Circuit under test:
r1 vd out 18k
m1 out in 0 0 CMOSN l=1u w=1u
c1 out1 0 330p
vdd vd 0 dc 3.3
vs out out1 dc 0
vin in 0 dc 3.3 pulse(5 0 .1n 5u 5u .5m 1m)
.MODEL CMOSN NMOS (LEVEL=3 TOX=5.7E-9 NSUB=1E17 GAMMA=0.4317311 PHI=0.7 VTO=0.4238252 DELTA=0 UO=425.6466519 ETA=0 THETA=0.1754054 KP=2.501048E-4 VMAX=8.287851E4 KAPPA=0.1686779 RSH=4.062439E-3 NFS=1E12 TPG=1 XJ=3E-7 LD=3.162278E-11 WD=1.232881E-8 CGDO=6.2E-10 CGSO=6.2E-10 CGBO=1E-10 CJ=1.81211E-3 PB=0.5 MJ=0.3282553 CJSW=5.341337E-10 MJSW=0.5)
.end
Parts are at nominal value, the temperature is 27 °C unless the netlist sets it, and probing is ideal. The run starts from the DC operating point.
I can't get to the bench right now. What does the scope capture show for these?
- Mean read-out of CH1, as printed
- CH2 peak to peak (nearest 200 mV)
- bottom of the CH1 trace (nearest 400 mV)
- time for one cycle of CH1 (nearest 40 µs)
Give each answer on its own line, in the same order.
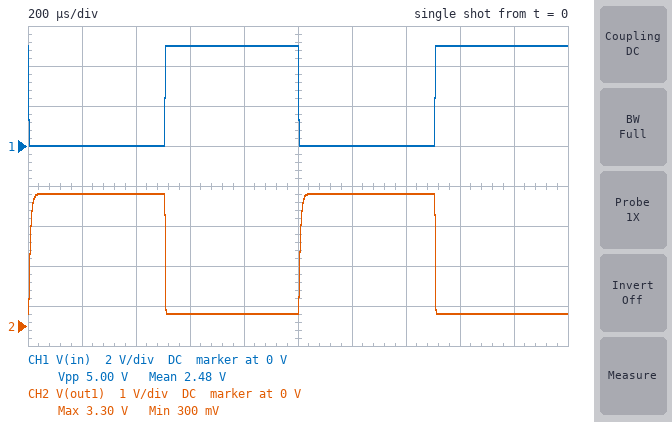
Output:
2.48 V
3.0 V
0 V
1.00 ms
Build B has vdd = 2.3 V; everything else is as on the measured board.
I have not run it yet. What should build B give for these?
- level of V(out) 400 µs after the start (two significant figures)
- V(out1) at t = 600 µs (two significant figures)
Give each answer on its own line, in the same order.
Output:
2.3 V
200 mV
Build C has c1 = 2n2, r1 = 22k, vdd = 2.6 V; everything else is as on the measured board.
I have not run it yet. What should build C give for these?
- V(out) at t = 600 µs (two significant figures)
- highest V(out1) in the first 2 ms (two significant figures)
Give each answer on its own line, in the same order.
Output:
190 mV
2.6 V
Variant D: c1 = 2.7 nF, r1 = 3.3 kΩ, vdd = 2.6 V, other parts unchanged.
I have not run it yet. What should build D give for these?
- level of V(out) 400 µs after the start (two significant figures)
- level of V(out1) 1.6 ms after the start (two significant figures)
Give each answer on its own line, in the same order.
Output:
2.6 V
1.1 V
